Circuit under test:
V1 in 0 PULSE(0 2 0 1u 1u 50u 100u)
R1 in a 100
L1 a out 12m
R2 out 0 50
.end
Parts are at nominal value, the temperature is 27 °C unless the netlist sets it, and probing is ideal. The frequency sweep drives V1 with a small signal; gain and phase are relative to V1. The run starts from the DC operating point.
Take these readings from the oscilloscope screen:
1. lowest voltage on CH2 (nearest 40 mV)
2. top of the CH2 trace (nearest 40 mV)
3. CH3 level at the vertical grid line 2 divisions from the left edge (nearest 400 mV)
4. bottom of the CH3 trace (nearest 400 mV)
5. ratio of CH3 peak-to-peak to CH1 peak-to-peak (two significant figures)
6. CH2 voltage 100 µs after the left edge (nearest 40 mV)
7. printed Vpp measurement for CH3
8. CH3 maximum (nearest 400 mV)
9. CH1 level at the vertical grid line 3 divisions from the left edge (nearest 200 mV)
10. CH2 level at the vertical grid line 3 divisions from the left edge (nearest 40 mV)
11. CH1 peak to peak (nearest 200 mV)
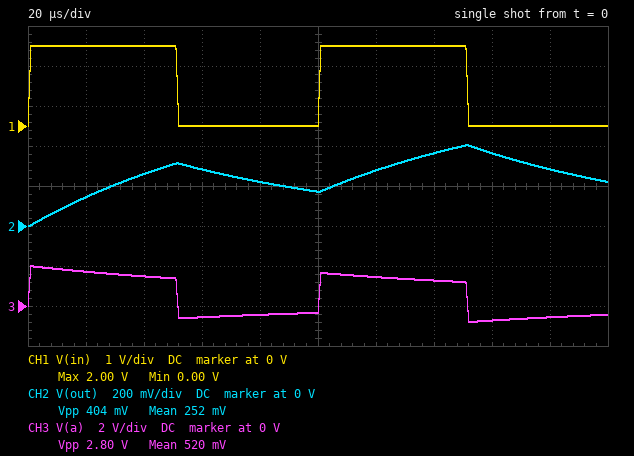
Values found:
0 V
400 mV
1.6 V
-800 mV
1.4
160 mV
2.80 V
2.0 V
0 V
280 mV
2.0 V
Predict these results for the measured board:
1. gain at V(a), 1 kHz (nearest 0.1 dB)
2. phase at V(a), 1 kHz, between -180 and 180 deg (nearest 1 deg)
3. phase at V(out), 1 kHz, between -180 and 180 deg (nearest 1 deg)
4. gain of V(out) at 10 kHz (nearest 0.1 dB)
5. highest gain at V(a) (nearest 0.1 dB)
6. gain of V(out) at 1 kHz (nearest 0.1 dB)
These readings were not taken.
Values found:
-5.4 dB
30 deg
-27 deg
-23.7 dB
0 dB
-10.5 dB
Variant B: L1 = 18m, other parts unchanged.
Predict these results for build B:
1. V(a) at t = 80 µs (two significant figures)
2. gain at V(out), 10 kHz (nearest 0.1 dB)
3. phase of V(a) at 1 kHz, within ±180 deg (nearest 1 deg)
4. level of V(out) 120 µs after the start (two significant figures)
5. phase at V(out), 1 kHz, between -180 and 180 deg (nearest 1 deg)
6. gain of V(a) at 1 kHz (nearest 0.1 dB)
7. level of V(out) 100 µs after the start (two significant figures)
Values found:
-360 mV
-27.2 dB
29 deg
230 mV
-37 deg
-3.6 dB
150 mV
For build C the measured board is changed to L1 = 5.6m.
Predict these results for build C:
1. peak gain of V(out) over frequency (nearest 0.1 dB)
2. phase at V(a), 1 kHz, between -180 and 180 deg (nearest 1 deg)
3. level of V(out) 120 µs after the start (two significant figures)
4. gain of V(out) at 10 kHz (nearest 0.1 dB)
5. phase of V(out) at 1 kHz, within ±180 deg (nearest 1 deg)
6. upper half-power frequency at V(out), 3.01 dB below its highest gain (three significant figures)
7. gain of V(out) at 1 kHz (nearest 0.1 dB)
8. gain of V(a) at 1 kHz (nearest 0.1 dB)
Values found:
-9.5 dB
22 deg
350 mV
-17.7 dB
-13 deg
4.26 kHz
-9.8 dB
-8.0 dB
